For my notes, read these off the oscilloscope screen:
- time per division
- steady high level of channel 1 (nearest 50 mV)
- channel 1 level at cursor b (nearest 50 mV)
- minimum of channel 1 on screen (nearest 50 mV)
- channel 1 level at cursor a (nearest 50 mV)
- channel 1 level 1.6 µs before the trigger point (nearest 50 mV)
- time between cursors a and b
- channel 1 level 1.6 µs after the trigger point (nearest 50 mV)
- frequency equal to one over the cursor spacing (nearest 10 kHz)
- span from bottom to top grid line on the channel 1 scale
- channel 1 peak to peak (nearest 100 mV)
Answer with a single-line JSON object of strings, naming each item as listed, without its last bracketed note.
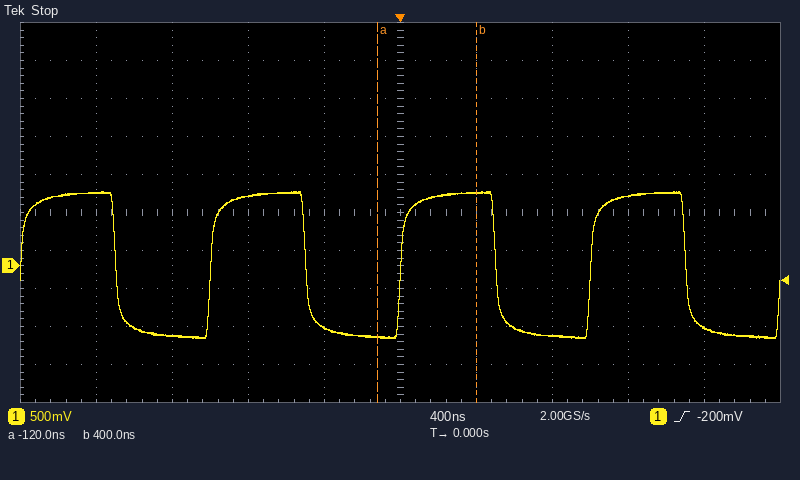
{"time per division": "400 ns", "steady high level of channel 1": "950 mV", "channel 1 level at cursor b": "950 mV", "minimum of channel 1 on screen": "-950 mV", "channel 1 level at cursor a": "-950 mV", "channel 1 level 1.6 µs before the trigger point": "950 mV", "time between cursors a and b": "520 ns", "channel 1 level 1.6 µs after the trigger point": "-800 mV", "frequency equal to one over the cursor spacing": "1.92 MHz", "span from bottom to top grid line on the channel 1 scale": "5 V", "channel 1 peak to peak": "1.90 V"}
